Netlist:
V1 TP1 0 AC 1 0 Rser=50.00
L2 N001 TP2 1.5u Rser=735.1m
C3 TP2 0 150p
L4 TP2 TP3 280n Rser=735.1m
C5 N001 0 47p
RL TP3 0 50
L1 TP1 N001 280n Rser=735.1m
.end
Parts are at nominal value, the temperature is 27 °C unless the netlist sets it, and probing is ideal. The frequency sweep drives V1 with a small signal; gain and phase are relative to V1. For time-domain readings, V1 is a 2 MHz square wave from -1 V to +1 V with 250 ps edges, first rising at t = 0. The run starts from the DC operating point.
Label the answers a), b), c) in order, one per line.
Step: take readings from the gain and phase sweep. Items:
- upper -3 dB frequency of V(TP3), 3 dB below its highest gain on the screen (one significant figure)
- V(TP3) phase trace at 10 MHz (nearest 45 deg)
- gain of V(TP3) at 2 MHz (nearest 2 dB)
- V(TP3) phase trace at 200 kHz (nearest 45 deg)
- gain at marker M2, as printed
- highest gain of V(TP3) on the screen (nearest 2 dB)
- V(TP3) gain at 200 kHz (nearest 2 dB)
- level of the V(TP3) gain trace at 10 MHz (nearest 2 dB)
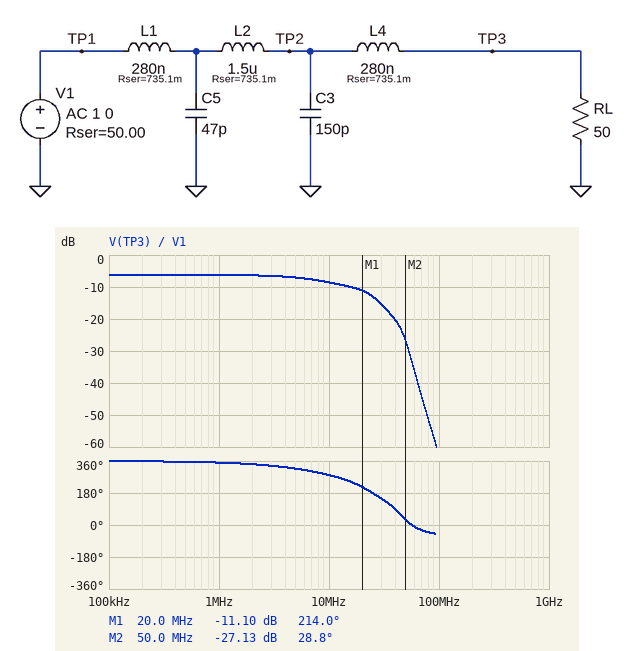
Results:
a) 10 MHz
b) 270 deg
c) -6 dB
d) 360 deg
e) -27.13 dB
f) -6 dB
g) -6 dB
h) -8 dB
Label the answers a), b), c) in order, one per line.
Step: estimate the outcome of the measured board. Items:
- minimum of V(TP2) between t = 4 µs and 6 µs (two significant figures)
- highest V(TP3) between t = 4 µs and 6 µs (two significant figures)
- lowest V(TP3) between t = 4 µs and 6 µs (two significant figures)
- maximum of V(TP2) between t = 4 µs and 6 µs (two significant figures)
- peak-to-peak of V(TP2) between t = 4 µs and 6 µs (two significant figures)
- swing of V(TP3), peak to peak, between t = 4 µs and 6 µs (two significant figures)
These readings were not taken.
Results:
a) -500 mV
b) 490 mV
c) -490 mV
d) 500 mV
e) 990 mV
f) 980 mV
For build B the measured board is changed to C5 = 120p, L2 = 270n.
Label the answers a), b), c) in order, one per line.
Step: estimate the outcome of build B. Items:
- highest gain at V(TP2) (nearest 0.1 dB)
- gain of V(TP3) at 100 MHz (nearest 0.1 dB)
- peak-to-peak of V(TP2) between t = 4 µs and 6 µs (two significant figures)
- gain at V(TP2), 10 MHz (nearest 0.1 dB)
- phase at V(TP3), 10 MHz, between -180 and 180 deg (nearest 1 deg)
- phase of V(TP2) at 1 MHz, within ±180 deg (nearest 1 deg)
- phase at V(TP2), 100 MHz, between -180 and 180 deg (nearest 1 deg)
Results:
a) -1.7 dB
b) -55.6 dB
c) 1.6 V
d) -5.6 dB
e) -55 deg
f) -3 deg
g) 19 deg
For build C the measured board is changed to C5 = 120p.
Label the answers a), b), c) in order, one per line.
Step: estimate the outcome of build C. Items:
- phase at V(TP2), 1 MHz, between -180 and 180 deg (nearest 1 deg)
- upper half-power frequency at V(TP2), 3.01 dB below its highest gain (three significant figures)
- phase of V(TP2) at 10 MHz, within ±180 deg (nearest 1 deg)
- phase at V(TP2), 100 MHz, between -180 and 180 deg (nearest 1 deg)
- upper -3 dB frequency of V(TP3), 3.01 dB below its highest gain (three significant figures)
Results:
a) -8 deg
b) 24.1 MHz
c) -70 deg
d) 18 deg
e) 17.7 MHz
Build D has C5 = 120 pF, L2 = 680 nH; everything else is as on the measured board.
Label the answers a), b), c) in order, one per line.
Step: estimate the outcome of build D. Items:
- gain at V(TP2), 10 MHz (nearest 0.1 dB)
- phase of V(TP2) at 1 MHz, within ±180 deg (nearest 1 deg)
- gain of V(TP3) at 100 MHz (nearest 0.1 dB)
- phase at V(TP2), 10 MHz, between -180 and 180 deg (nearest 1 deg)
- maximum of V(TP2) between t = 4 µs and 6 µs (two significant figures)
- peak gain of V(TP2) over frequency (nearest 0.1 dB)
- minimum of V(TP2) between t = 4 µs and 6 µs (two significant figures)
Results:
a) -5.8 dB
b) -5 deg
c) -64.5 dB
d) -48 deg
e) 730 mV
f) -4.0 dB
g) -730 mV
